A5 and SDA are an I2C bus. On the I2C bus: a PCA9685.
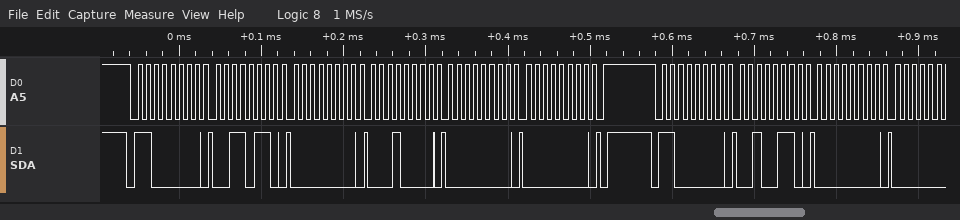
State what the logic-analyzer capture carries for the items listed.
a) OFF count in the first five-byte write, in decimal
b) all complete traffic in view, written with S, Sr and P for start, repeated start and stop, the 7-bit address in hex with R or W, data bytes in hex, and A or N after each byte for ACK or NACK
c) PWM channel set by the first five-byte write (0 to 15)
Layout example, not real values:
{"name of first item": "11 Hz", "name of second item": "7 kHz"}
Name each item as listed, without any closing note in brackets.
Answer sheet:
{"OFF count in the first five-byte write, in decimal": "0", "all complete traffic in view, written with S, Sr and P for start, repeated start and stop, the 7-bit address in hex with R or W, data bytes in hex, and A or N after each byte for ACK or NACK": "S 60W A 36 A 00 A 10 A 00 A 00 A P S 60W A 26 A 00 A", "PWM channel set by the first five-byte write": "12"}
